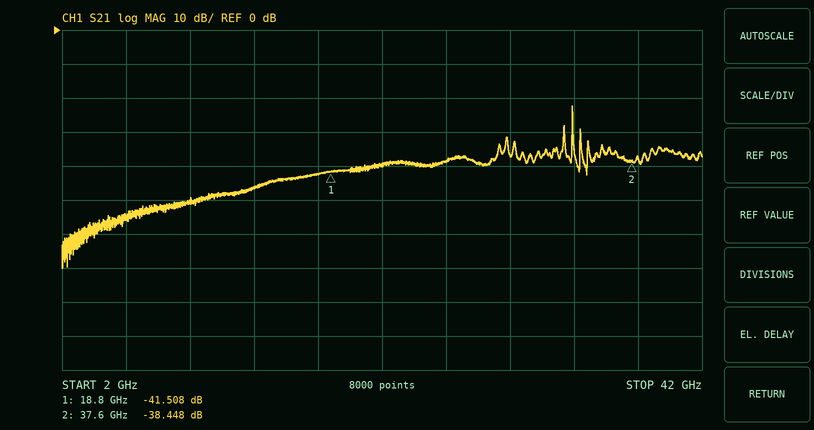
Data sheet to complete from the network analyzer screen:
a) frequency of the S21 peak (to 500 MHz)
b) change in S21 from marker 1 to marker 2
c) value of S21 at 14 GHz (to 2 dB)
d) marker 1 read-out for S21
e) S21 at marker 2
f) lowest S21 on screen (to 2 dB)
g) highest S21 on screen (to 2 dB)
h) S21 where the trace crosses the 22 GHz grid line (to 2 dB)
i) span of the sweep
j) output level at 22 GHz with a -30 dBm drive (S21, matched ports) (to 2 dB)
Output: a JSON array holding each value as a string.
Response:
["34.0 GHz", "3.060 dB", "-46 dB", "-41.508 dB", "-38.448 dB", "-70 dB", "-22 dB", "-40 dB", "40 GHz", "-70 dBm"]
